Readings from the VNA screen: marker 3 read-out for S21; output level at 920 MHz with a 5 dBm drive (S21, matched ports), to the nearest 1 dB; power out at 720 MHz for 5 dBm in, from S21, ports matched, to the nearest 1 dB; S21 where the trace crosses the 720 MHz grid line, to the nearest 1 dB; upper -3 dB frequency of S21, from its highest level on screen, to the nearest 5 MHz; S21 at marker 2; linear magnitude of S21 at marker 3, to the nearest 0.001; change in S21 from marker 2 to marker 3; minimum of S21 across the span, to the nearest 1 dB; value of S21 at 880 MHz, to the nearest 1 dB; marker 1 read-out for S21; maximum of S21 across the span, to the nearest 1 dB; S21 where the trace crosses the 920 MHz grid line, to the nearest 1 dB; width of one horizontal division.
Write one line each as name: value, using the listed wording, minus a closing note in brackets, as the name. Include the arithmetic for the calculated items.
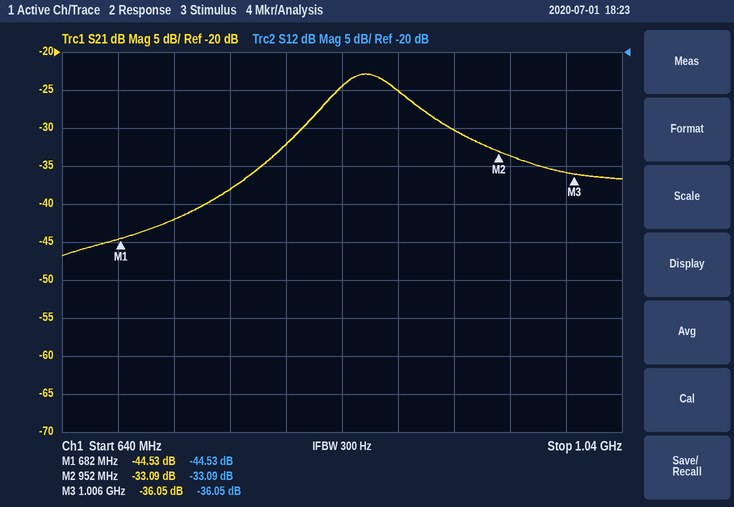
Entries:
marker 3 read-out for S21: -36.05 dB
output level at 920 MHz with a 5 dBm drive (S21, matched ports), to the nearest 1 dB: 5 dBm + (-30 dB) = -25 dBm
power out at 720 MHz for 5 dBm in, from S21, ports matched, to the nearest 1 dB: 5 dBm + (-42 dB) = -37 dBm
S21 where the trace crosses the 720 MHz grid line, to the nearest 1 dB: -42 dB
upper -3 dB frequency of S21, from its highest level on screen, to the nearest 5 MHz: 885 MHz
S21 at marker 2: -33.09 dB
linear magnitude of S21 at marker 3, to the nearest 0.001: 10^(-36.05/20) ≈ 0.016
change in S21 from marker 2 to marker 3: -36.05 − (-33.09) = -2.96 dB
minimum of S21 across the span, to the nearest 1 dB: -47 dB
value of S21 at 880 MHz, to the nearest 1 dB: -25 dB
marker 1 read-out for S21: -44.53 dB
maximum of S21 across the span, to the nearest 1 dB: -23 dB
S21 where the trace crosses the 920 MHz grid line, to the nearest 1 dB: -30 dB
width of one horizontal division: 40 MHz
